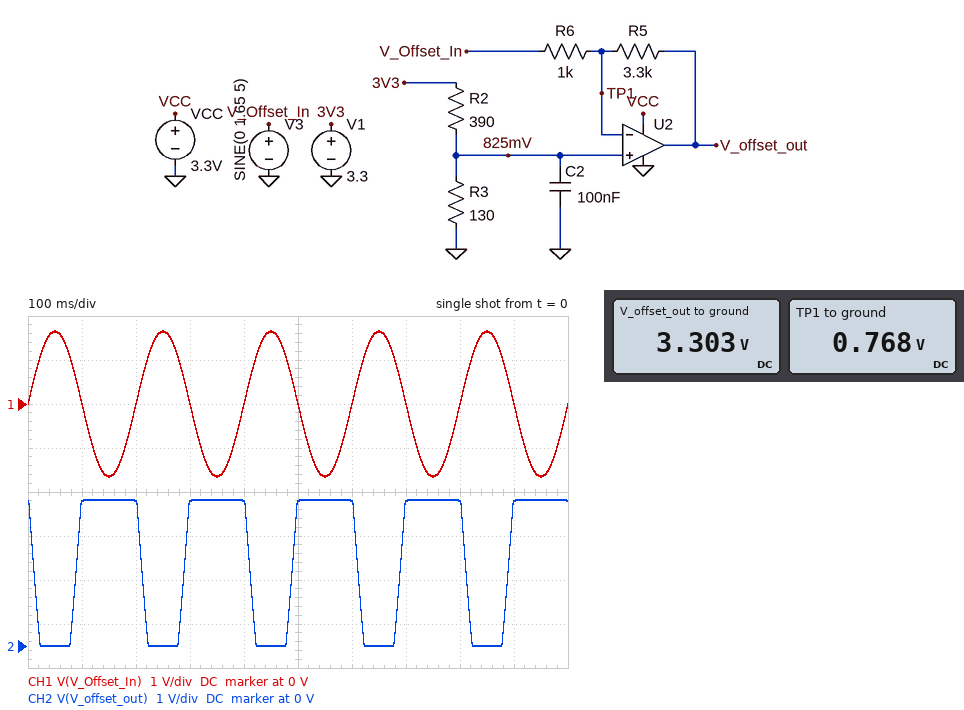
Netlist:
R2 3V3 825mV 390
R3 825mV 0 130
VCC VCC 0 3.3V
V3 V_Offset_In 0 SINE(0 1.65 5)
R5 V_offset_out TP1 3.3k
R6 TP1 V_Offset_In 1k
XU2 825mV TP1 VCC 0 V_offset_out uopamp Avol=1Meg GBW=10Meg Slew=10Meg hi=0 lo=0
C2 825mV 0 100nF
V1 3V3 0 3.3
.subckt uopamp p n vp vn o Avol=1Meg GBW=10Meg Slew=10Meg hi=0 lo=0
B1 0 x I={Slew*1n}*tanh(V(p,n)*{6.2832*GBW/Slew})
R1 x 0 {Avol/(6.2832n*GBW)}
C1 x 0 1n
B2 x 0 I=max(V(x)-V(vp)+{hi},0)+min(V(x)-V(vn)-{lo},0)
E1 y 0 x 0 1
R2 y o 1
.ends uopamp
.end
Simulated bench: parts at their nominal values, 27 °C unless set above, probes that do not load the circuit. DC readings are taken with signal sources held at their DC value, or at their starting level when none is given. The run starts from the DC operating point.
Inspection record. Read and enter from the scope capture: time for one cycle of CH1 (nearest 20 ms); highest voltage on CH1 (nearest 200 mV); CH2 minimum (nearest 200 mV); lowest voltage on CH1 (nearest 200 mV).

200 ms
1.6 V
0 V
-1.6 V
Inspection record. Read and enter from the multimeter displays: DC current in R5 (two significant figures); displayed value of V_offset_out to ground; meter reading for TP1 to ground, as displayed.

770 µA
3.303 V
0.768 V
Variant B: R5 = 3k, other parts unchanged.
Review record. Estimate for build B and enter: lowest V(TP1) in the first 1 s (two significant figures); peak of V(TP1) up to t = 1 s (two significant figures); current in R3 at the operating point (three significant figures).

-410 mV
1.2 V
6.35 mA
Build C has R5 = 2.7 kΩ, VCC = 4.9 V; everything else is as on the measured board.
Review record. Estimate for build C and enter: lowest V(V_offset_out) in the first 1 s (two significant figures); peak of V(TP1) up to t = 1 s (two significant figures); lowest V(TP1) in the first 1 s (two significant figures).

-9.4 mV
1.2 V
120 mV
